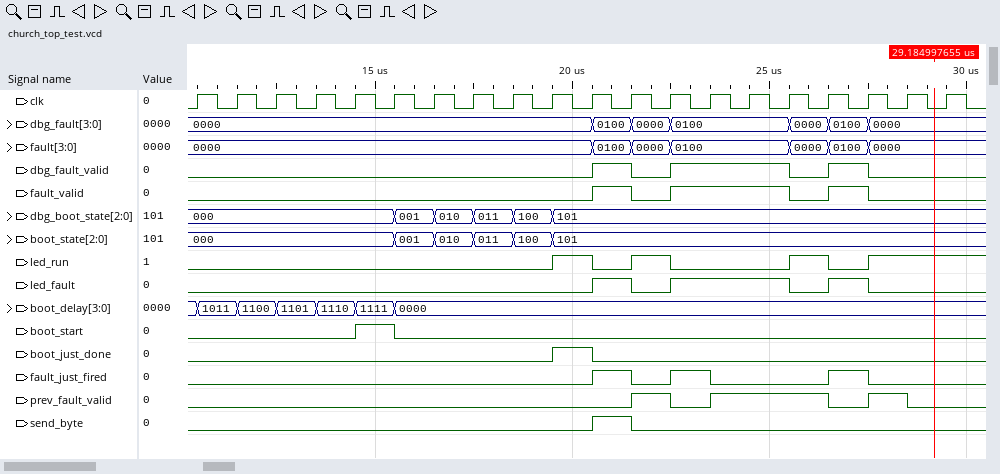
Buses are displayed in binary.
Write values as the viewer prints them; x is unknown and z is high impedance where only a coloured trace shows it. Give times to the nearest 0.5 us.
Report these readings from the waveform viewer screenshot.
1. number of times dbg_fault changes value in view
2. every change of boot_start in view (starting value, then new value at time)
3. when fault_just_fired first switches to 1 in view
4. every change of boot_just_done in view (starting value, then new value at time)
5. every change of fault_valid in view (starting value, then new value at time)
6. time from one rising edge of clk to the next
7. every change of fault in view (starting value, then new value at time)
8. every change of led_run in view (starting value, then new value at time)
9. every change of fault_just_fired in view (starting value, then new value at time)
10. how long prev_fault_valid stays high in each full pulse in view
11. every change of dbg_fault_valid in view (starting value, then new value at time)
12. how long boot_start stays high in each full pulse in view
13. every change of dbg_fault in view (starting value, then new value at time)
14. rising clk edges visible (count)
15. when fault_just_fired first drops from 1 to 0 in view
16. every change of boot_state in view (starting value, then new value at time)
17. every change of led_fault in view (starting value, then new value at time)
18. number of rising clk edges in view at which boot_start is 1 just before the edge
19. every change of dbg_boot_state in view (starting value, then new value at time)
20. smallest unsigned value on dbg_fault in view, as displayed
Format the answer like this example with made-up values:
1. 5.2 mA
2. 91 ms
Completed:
1. 6
2. 0, 1 at 14.5 us, 0 at 15.5 us
3. 20.5 us
4. 0, 1 at 19.5 us, 0 at 20.5 us
5. 0, 1 at 20.5 us, 0 at 21.5 us, 1 at 22.5 us, 0 at 25.5 us, 1 at 26.5 us, 0 at 27.5 us
6. 1 us
7. 0000, 0100 at 20.5 us, 0000 at 21.5 us, 0100 at 22.5 us, 0000 at 25.5 us, 0100 at 26.5 us, 0000 at 27.5 us
8. 0, 1 at 19.5 us, 0 at 20.5 us, 1 at 21.5 us, 0 at 22.5 us, 1 at 25.5 us, 0 at 26.5 us, 1 at 27.5 us
9. 0, 1 at 20.5 us, 0 at 21.5 us, 1 at 22.5 us, 0 at 23.5 us, 1 at 26.5 us, 0 at 27.5 us
10. 1 us, 3 us, 1 us
11. 0, 1 at 20.5 us, 0 at 21.5 us, 1 at 22.5 us, 0 at 25.5 us, 1 at 26.5 us, 0 at 27.5 us
12. 1 us
13. 0000, 0100 at 20.5 us, 0000 at 21.5 us, 0100 at 22.5 us, 0000 at 25.5 us, 0100 at 26.5 us, 0000 at 27.5 us
14. 20
15. 21.5 us
16. 000, 001 at 15.5 us, 010 at 16.5 us, 011 at 17.5 us, 100 at 18.5 us, 101 at 19.5 us
17. 0, 1 at 20.5 us, 0 at 21.5 us, 1 at 22.5 us, 0 at 25.5 us, 1 at 26.5 us, 0 at 27.5 us
18. 1
19. 000, 001 at 15.5 us, 010 at 16.5 us, 011 at 17.5 us, 100 at 18.5 us, 101 at 19.5 us
20. 0000
